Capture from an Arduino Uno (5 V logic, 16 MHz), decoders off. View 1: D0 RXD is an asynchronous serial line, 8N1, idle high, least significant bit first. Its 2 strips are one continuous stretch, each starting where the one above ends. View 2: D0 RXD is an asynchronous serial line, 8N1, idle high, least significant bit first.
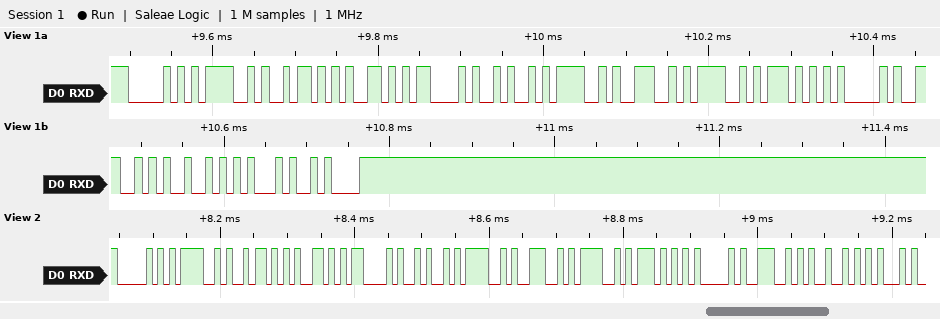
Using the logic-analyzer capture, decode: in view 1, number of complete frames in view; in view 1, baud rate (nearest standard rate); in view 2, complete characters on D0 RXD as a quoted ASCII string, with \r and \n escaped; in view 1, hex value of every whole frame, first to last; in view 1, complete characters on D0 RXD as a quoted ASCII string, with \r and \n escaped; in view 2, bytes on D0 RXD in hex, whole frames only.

15
115200 baud
"POZYCJONOWANIE"
50 4F 5A 59 43 4A 4F 4E 4F 57 41 4E 49 45 0A
"POZYCJONOWANIE\n"
50 4F 5A 59 43 4A 4F 4E 4F 57 41 4E 49 45
